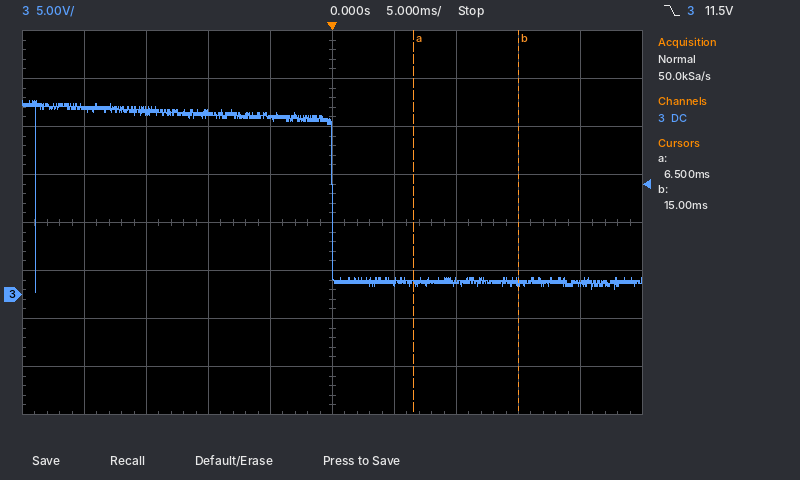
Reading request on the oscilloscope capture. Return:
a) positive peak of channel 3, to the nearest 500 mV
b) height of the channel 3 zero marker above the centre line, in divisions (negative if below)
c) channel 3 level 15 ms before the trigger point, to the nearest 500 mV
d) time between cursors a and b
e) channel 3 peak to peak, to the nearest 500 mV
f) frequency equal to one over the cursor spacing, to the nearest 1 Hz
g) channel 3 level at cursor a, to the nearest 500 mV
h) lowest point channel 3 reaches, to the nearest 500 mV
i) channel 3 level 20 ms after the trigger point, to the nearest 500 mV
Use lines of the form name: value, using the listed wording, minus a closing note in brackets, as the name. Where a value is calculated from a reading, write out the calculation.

positive peak of channel 3, to the nearest 500 mV: 20.0 V
height of the channel 3 zero marker above the centre line, in divisions: -1.5 div
channel 3 level 15 ms before the trigger point, to the nearest 500 mV: 19.0 V
time between cursors a and b: 15 ms − (6.5 ms) = 8.5 ms
channel 3 peak to peak, to the nearest 500 mV: 20.0 V − (0.0 V) = 20.0 V
frequency equal to one over the cursor spacing, to the nearest 1 Hz: 1 / 8.5 ms ≈ 118 Hz
channel 3 level at cursor a, to the nearest 500 mV: 1.0 V
lowest point channel 3 reaches, to the nearest 500 mV: 0.0 V
channel 3 level 20 ms after the trigger point, to the nearest 500 mV: 1.0 V
